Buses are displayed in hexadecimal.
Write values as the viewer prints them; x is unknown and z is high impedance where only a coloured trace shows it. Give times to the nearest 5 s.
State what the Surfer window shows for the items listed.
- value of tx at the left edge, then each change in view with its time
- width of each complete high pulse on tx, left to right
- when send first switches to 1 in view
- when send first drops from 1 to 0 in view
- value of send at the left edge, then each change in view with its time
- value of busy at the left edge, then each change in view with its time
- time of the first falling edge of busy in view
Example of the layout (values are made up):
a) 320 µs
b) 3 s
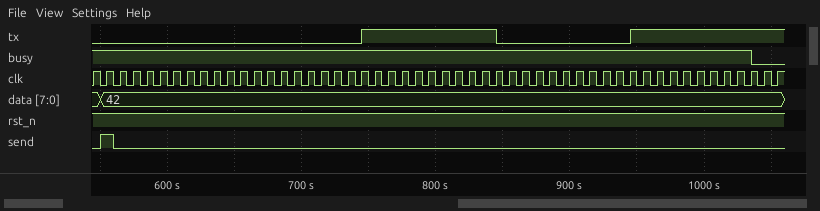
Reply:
a) 0, 1 at 745 s, 0 at 845 s, 1 at 945 s
b) 100 s
c) 550 s
d) 560 s
e) 0, 1 at 550 s, 0 at 560 s
f) 1, 0 at 1035 s
g) 1035 s
